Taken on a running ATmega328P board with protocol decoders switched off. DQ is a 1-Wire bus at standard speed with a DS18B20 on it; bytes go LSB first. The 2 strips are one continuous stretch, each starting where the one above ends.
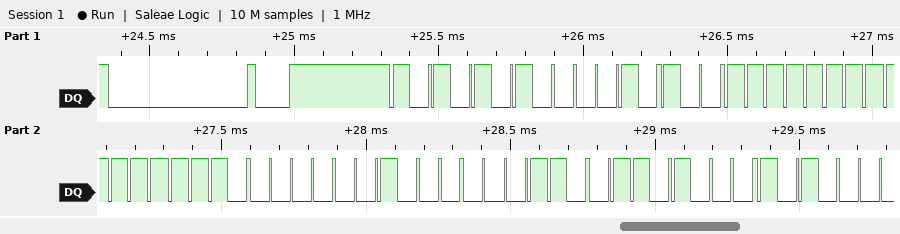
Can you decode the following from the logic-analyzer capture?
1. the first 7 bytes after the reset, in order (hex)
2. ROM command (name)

55 28 FF 7F 40 60 16
Match ROM
